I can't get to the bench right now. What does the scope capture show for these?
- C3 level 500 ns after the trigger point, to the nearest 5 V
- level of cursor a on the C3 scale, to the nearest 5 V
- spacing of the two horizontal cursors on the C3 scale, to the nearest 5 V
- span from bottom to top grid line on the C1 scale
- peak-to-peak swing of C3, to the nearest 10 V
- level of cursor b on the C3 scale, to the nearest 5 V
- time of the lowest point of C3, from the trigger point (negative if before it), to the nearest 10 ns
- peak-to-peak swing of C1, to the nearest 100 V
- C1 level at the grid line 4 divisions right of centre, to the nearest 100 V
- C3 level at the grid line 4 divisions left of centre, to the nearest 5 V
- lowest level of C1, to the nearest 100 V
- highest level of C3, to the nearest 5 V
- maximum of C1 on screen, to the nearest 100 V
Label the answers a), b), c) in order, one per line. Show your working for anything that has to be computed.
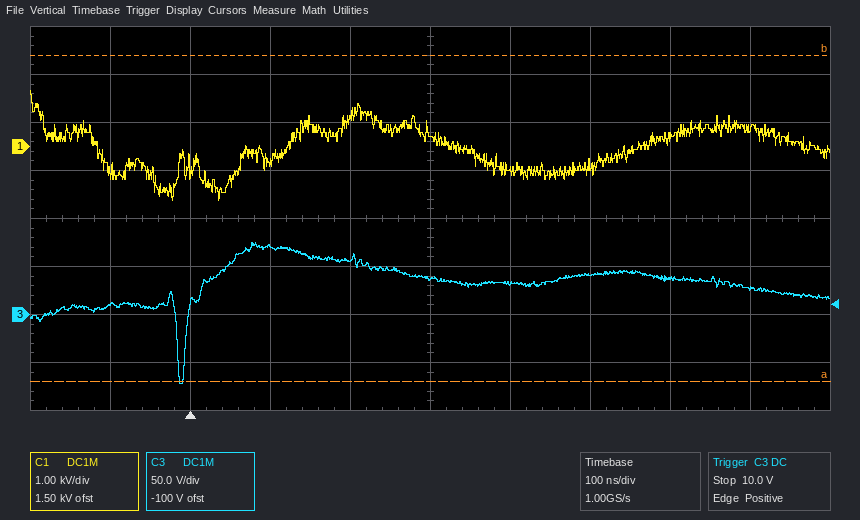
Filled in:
a) 40 V
b) -70 V
c) 340 V
d) 8 kV
e) 150 V
f) 270 V
g) -10 ns
h) 1.2 kV − (-1.1 kV) = 2.3 kV
i) 400 V
j) 10 V
k) -1.1 kV
l) 75 V
m) 1.2 kV
